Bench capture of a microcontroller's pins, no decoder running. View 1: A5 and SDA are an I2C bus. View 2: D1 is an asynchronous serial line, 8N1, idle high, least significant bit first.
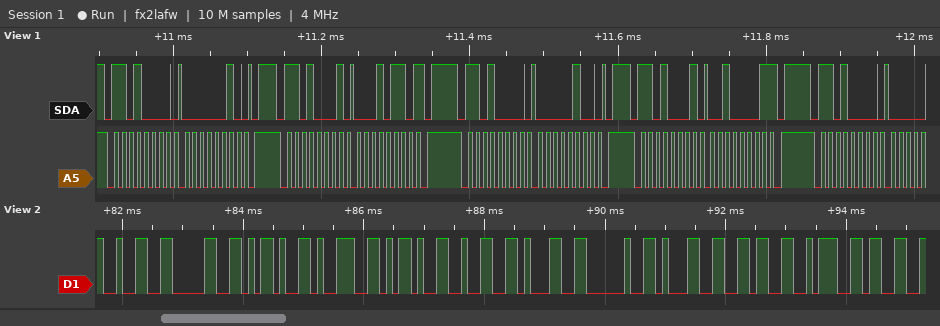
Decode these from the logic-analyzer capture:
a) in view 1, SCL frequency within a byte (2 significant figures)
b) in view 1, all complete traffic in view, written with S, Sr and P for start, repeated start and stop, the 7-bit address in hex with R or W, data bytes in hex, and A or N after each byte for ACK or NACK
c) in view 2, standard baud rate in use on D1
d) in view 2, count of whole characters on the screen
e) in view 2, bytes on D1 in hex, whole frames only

100 kHz
S 68W A 02 A P S 68R A 16 N P S 68W A 04 A P S 68R A 21 N P S 68W A
9600 baud
12
0x32 0x30 0x2D 0x39 0x2D 0x32 0x31 0x20 0x31 0x36 0x3A 0x33
